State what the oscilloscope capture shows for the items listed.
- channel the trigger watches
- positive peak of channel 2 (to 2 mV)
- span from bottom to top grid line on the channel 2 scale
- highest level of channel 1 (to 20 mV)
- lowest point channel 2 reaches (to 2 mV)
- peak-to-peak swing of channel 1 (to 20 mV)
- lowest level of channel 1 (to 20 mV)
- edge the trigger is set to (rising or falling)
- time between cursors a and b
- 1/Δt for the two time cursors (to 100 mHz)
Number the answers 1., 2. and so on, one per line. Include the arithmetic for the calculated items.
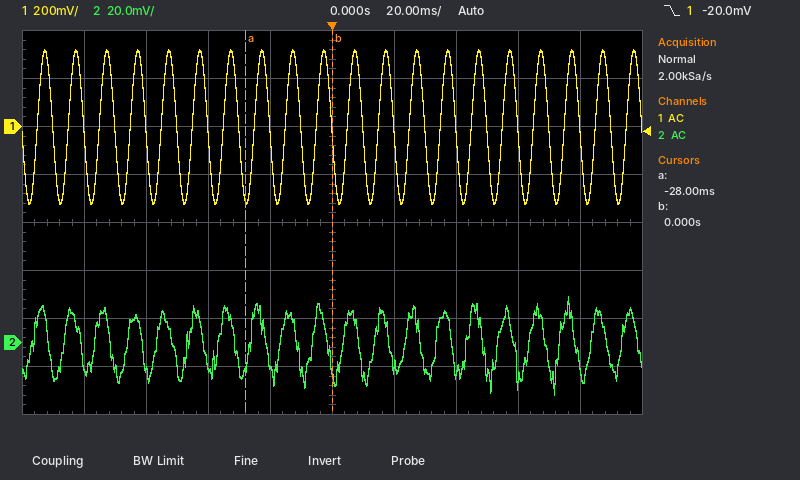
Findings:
1. channel 1
2. 20 mV
3. 160 mV
4. 320 mV
5. -22 mV
6. 320 mV − (-320 mV) = 640 mV
7. -320 mV
8. falling
9. 0 s − (-28 ms) = 28 ms
10. 1 / 28 ms ≈ 35.7 Hz
